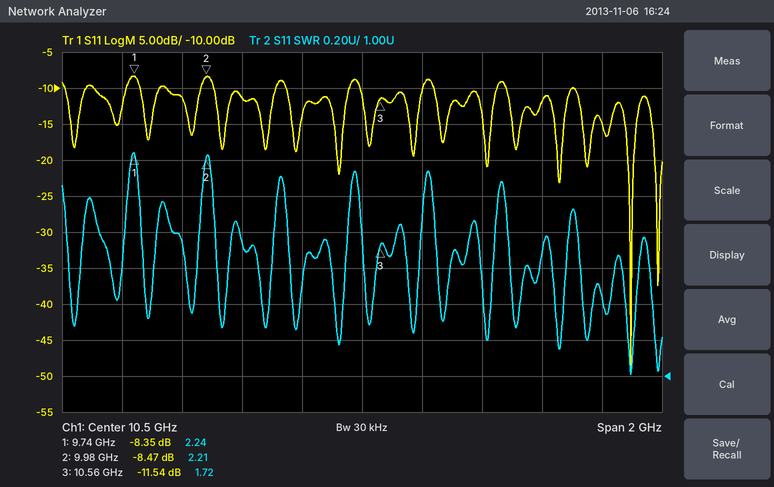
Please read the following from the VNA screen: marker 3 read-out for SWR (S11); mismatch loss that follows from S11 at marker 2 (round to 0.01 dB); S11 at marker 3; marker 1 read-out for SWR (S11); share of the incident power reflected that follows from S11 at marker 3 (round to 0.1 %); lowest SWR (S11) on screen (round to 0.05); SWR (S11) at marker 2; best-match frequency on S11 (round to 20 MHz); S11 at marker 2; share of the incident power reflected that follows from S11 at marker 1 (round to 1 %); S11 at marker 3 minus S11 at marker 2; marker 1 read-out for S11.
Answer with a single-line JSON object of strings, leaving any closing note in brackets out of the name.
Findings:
{"marker 3 read-out for SWR": "1.72", "mismatch loss that follows from S11 at marker 2": "0.67 dB", "S11 at marker 3": "-11.54 dB", "marker 1 read-out for SWR": "2.24", "share of the incident power reflected that follows from S11 at marker 3": "7.0 %", "lowest SWR (S11) on screen": "1.00", "SWR (S11) at marker 2": "2.21", "best-match frequency on S11": "11.40 GHz", "S11 at marker 2": "-8.47 dB", "share of the incident power reflected that follows from S11 at marker 1": "15 %", "S11 at marker 3 minus S11 at marker 2": "-3.07 dB", "marker 1 read-out for S11": "-8.35 dB"}
